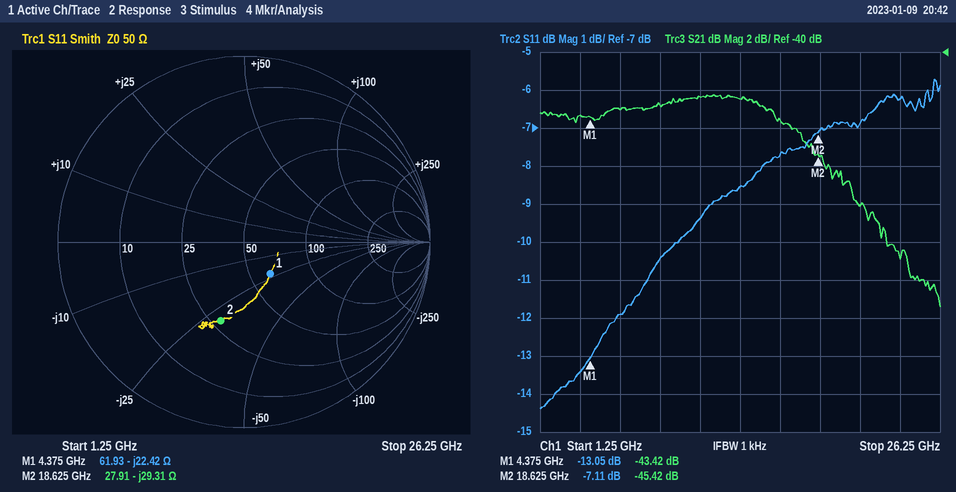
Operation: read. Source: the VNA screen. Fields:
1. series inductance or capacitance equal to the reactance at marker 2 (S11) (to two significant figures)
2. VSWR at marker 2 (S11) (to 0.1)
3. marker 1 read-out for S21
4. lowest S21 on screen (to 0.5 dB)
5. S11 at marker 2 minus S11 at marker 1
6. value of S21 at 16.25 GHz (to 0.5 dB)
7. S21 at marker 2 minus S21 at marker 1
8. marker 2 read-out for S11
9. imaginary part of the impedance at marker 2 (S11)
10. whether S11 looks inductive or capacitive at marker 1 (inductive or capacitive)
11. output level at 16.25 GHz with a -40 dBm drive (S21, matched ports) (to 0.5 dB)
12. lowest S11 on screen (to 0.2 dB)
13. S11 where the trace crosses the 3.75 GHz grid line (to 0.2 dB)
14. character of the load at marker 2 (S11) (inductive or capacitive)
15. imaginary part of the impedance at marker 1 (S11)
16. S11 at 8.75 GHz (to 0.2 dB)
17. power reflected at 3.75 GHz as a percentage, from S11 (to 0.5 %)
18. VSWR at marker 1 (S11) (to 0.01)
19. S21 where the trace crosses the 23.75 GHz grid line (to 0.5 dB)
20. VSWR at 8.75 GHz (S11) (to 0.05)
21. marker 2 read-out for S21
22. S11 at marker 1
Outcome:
290 fF
2.6
-43.42 dB
-53.5 dB
5.94 dB
-43.5 dB
-2.00 dB
-7.11 dB
-29.31 Ω
capacitive
-83.5 dBm
-14.4 dB
-13.4 dB
capacitive
-22.42 Ω
-10.4 dB
4.5 %
1.57
-51.0 dB
1.85
-45.42 dB
-13.05 dB
